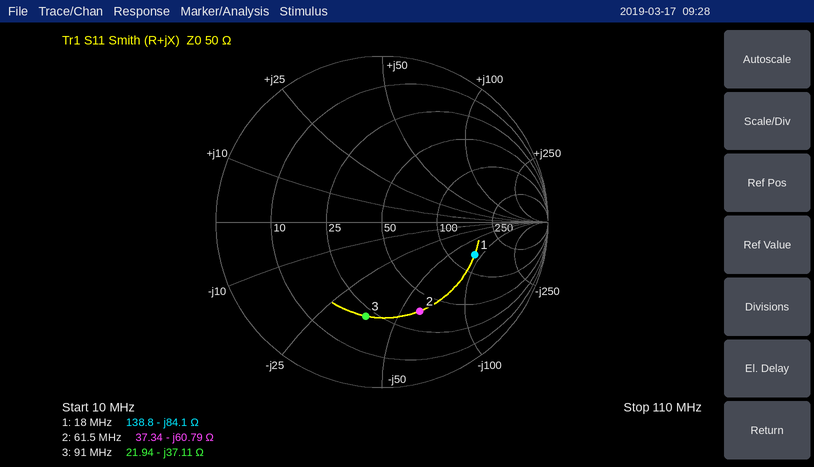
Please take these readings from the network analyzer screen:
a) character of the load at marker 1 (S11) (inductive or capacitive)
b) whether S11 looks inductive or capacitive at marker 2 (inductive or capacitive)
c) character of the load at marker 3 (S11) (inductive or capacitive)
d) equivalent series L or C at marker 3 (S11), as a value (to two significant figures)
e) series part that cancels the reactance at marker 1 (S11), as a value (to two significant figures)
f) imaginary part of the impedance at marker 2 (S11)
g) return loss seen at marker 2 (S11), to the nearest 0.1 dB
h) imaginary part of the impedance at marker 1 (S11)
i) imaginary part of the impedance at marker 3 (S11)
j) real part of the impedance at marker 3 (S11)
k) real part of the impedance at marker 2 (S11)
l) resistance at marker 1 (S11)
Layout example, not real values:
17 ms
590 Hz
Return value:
capacitive
capacitive
capacitive
47 pF
740 nH
-60.79 Ω
4.7 dB
-84.1 Ω
-37.11 Ω
21.94 Ω
37.34 Ω
138.8 Ω
